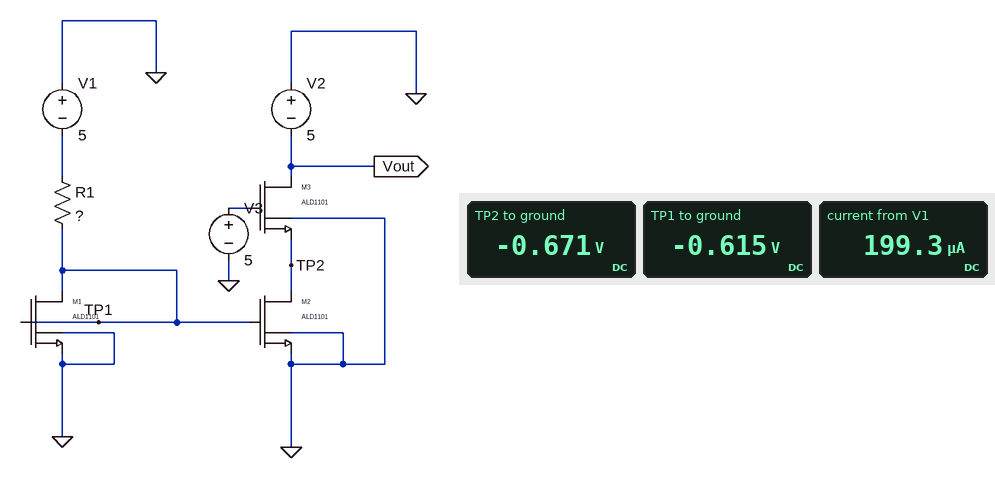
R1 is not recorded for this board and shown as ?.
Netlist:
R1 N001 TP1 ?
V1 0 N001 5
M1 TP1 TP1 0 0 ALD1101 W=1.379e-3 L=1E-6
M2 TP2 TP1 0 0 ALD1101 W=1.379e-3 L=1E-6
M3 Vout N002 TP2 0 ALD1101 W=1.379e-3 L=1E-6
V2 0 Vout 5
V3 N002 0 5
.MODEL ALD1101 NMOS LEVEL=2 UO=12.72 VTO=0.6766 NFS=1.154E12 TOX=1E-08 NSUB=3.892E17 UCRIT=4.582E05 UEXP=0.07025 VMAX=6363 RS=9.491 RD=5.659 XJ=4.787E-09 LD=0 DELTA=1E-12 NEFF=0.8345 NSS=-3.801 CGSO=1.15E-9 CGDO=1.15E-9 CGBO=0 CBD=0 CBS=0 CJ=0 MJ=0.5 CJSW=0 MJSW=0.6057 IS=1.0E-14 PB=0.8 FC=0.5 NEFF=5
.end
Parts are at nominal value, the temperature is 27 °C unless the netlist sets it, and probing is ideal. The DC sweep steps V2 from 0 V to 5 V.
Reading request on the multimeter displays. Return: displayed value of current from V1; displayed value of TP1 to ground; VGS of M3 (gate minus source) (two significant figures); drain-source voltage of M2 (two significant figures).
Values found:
199.3 µA
-0.615 V
5.7 V
-670 mV
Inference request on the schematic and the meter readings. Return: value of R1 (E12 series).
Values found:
22 kΩ
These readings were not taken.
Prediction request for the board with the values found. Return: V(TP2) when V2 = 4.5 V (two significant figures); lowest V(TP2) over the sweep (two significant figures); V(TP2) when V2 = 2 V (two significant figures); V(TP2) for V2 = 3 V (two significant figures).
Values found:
-670 mV
-670 mV
-670 mV
-670 mV
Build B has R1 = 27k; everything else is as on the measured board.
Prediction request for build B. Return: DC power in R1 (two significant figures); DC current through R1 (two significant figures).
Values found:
710 µW
160 µA
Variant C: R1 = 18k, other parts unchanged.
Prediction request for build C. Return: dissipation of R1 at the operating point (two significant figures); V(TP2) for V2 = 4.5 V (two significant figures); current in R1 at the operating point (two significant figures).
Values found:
1.1 mW
-670 mV
240 µA
